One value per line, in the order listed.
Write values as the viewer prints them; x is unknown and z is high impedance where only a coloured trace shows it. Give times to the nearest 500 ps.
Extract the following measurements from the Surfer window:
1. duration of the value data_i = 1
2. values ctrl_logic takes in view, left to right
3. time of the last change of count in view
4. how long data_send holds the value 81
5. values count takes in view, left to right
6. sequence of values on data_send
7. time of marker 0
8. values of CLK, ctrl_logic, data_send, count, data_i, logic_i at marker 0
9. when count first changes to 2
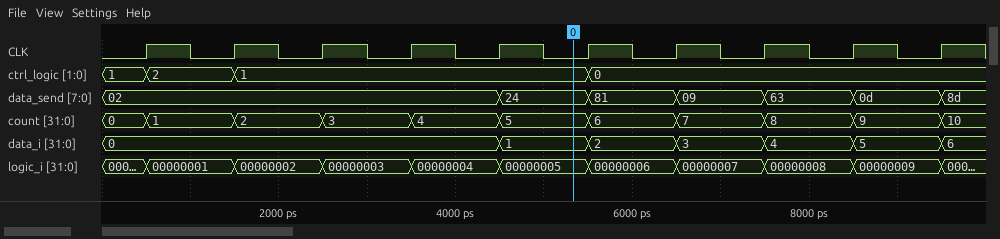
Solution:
1000 ps
1, 2, 1, 0
9500 ps
1000 ps
0, 1, 2, 3, 4, 5, 6, 7, 8, 9, 10
02, 24, 81, 09, 63, 0d, 8d
5500 ps
CLK=0, ctrl_logic=1, data_send=24, count=5, data_i=1, logic_i=00000005
1500 ps
